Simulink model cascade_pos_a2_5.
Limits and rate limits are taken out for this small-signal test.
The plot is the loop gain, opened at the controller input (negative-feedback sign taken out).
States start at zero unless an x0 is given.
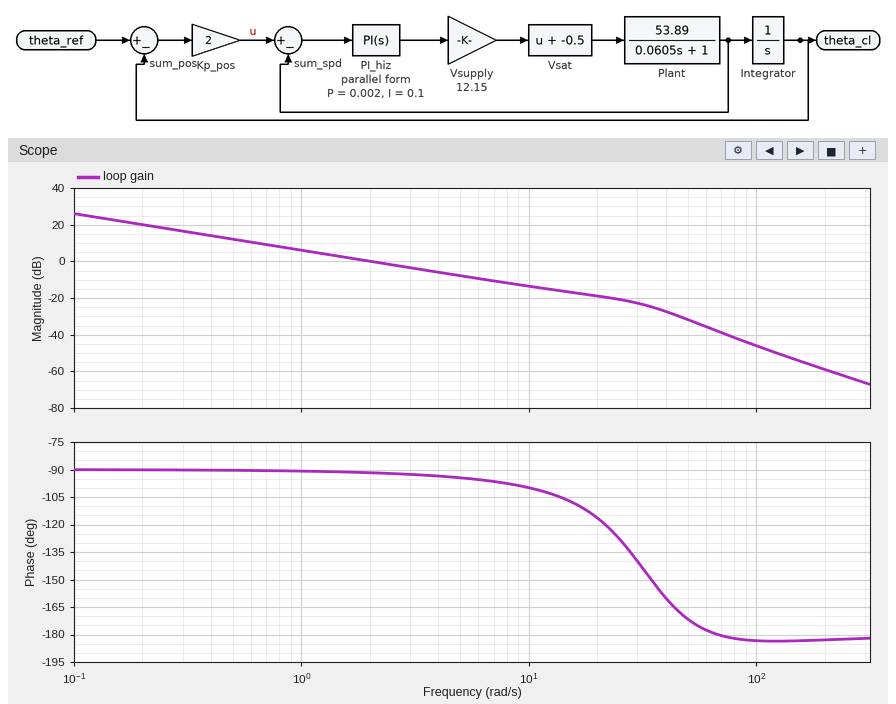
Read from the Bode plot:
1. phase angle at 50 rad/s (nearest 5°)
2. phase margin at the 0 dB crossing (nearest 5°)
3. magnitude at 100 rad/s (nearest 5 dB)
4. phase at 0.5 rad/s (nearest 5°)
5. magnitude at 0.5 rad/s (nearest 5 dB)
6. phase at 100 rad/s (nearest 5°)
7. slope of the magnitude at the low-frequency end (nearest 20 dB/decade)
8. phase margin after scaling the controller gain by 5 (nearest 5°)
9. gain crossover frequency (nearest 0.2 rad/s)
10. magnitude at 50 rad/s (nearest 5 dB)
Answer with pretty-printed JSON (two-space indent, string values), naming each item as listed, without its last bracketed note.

{
  "phase angle at 50 rad/s": "-170°",
  "phase margin at the 0 dB crossing": "90°",
  "magnitude at 100 rad/s": "-45 dB",
  "phase at 0.5 rad/s": "-90°",
  "magnitude at 0.5 rad/s": "10 dB",
  "phase at 100 rad/s": "-185°",
  "slope of the magnitude at the low-frequency end": "-20 dB/decade",
  "phase margin after scaling the controller gain by 5": "80°",
  "gain crossover frequency": "2.0 rad/s",
  "magnitude at 50 rad/s": "-30 dB"
}
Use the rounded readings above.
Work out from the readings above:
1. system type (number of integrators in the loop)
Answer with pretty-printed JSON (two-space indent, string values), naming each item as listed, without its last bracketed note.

{
  "system type": "1"
}
